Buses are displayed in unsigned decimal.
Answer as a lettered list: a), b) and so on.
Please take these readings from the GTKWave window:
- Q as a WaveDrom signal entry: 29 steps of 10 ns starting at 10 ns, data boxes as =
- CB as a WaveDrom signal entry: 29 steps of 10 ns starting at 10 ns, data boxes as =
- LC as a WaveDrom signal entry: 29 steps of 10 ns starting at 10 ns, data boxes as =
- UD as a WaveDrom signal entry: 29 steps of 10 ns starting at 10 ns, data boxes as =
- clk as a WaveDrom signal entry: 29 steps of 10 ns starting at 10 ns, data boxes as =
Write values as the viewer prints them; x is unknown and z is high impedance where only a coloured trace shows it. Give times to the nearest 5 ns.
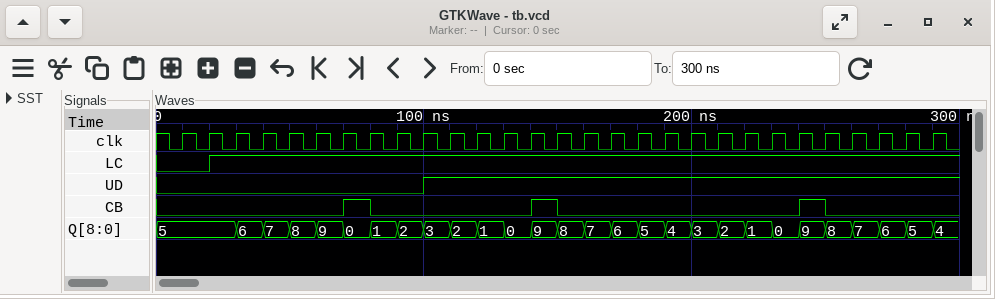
a) {name: 'Q', wave: '=.===========================', data: '5 6 7 8 9 0 1 2 3 2 1 0 9 8 7 6 5 4 3 2 1 0 9 8 7 6 5 4'}
b) {name: 'CB', wave: '0.....10.....10........10....'}
c) {name: 'LC', wave: '01...........................'}
d) {name: 'UD', wave: '0........1...................'}
e) {name: 'clk', wave: 'p............................'}
